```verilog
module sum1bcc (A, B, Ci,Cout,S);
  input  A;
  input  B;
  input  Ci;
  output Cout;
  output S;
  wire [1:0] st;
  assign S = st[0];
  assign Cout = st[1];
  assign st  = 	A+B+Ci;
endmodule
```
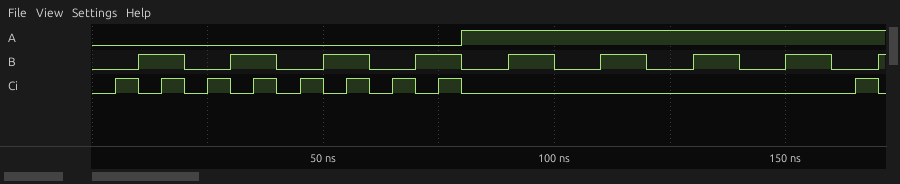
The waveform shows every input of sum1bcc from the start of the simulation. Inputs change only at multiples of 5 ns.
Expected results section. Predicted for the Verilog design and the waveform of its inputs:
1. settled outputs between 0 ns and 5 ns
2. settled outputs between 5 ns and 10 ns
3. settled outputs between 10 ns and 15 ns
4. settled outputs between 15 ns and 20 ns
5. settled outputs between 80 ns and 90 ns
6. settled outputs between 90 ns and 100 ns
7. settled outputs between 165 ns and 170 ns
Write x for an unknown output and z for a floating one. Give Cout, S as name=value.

Cout=0, S=0
Cout=0, S=1
Cout=0, S=1
Cout=1, S=0
Cout=0, S=1
Cout=1, S=0
Cout=1, S=0
